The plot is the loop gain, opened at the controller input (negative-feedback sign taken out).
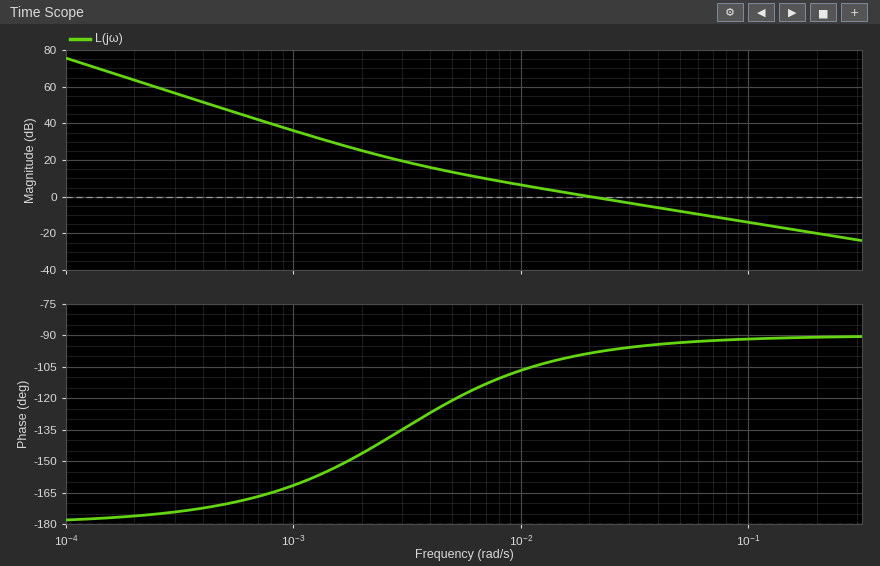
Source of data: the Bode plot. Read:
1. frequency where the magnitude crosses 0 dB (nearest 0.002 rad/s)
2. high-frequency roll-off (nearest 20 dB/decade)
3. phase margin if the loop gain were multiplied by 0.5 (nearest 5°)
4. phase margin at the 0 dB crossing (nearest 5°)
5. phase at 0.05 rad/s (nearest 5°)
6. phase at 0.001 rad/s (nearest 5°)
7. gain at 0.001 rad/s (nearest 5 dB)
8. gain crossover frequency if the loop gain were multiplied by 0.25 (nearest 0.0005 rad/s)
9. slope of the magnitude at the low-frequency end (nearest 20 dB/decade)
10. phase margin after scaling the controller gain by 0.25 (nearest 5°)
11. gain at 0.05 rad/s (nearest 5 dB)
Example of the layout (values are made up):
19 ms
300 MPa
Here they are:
0.020 rad/s
-20 dB/decade
75°
80°
-95°
-160°
35 dB
0.0055 rad/s
-40 dB/decade
60°
-10 dB
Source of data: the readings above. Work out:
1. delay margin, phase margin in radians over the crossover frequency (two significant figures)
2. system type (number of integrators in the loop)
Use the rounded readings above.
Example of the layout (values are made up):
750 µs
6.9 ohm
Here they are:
70 s
2
